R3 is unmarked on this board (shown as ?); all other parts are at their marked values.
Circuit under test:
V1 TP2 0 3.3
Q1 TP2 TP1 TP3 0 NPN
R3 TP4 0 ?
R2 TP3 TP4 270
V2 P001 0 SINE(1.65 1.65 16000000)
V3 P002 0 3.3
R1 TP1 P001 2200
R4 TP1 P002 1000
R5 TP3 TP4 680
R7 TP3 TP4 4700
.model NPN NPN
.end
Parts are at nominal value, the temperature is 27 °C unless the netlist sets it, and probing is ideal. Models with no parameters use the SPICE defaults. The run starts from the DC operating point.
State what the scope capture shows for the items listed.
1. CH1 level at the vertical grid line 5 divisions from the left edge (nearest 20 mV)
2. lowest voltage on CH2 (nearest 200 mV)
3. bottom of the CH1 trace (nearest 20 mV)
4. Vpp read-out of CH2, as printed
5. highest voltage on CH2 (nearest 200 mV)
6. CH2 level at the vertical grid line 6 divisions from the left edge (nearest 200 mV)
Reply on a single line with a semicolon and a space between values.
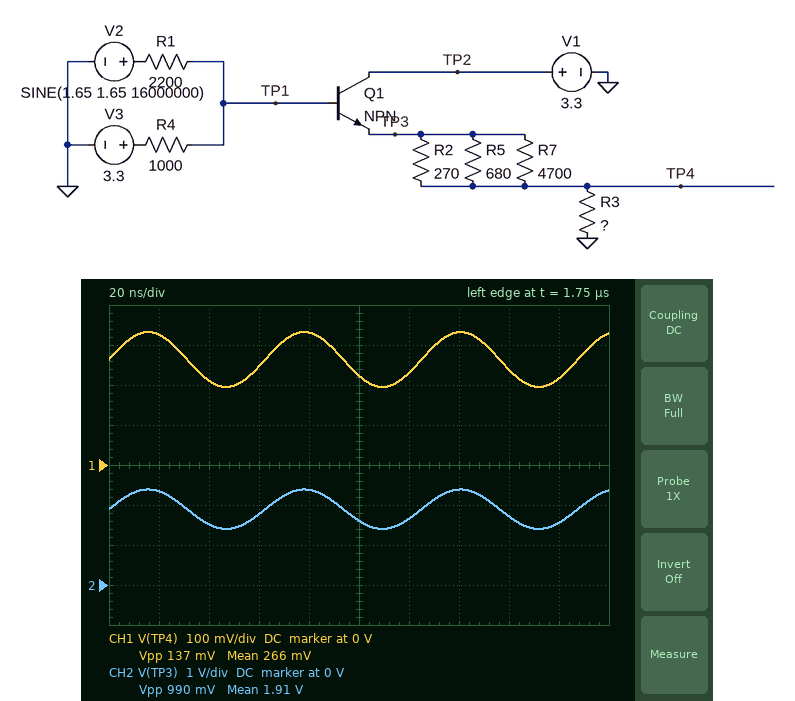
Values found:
220 mV; 1.4 V; 200 mV; 990 mV; 2.4 V; 1.6 V
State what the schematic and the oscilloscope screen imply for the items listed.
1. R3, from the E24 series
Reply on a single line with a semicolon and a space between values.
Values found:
30 Ω
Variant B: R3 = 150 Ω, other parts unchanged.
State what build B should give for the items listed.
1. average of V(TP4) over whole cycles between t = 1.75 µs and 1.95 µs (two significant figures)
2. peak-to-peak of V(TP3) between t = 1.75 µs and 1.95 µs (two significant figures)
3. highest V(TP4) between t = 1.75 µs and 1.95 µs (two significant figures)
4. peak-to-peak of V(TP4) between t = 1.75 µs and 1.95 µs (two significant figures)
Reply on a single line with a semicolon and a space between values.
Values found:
860 mV; 1.0 V; 1.1 V; 450 mV
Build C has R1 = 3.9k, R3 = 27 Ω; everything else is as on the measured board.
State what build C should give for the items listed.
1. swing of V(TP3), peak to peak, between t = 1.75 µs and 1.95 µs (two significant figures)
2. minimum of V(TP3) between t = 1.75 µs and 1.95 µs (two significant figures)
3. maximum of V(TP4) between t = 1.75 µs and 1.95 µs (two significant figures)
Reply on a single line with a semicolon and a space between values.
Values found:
640 mV; 1.7 V; 300 mV
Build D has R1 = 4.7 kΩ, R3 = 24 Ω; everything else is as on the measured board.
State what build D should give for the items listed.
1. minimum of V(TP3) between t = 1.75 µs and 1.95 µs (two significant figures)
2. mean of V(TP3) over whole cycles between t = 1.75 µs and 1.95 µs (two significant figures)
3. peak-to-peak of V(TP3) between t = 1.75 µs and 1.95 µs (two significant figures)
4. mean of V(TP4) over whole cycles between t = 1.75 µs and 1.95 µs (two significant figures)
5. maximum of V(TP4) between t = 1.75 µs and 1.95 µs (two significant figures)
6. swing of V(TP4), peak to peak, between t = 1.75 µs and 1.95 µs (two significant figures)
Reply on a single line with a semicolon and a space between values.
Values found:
1.8 V; 2.1 V; 550 mV; 240 mV; 270 mV; 63 mV
